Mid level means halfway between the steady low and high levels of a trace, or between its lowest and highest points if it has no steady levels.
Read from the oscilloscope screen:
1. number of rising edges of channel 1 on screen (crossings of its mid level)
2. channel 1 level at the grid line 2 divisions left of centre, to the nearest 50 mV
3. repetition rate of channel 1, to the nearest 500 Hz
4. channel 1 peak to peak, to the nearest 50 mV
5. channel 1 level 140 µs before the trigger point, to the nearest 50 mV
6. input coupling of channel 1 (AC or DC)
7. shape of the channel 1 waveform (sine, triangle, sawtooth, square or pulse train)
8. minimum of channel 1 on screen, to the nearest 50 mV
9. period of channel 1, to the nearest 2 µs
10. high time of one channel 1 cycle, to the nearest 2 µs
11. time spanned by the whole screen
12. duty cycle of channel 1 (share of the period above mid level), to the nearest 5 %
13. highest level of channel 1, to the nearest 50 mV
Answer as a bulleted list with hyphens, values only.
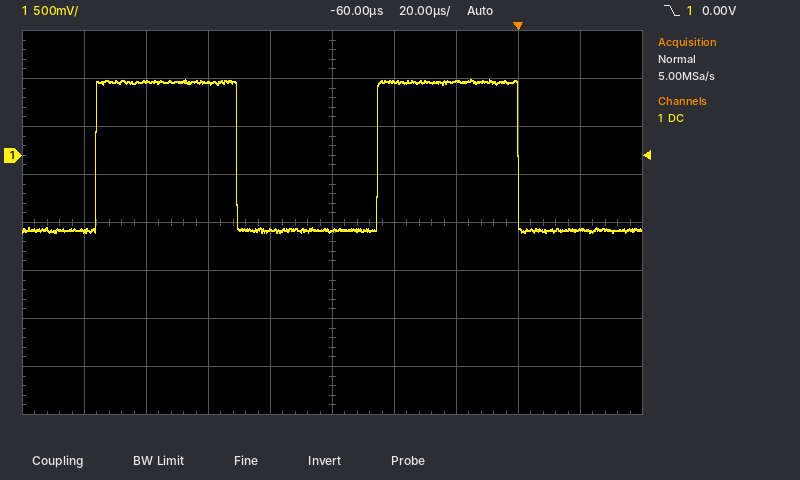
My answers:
- 2
- 750 mV
- 11.0 kHz
- 1.60 V
- -800 mV
- DC
- square
- -800 mV
- 90 µs
- 46 µs
- 200 µs
- 50 %
- 800 mV
